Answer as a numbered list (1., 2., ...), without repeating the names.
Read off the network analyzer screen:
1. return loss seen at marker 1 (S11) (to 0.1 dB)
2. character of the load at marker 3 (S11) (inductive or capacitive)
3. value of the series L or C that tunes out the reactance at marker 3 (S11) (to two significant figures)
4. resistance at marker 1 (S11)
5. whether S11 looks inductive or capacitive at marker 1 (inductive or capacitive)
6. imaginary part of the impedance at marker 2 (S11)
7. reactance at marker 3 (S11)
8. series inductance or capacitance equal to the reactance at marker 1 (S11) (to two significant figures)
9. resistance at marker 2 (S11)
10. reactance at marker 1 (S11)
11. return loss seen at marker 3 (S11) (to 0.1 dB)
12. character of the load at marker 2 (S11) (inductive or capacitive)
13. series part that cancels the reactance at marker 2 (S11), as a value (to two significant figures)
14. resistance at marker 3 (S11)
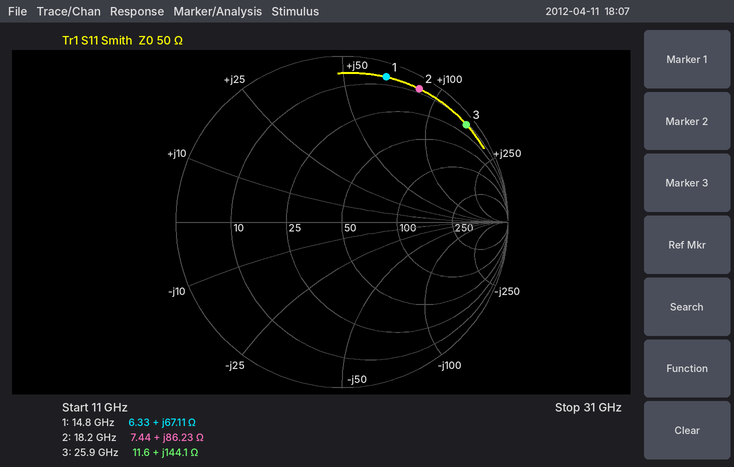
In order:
1. 0.8 dB
2. inductive
3. 43 fF
4. 6.33 Ω
5. inductive
6. +86.23 Ω
7. +144.1 Ω
8. 720 pH
9. 7.44 Ω
10. +67.11 Ω
11. 0.4 dB
12. inductive
13. 100 fF
14. 11.6 Ω
